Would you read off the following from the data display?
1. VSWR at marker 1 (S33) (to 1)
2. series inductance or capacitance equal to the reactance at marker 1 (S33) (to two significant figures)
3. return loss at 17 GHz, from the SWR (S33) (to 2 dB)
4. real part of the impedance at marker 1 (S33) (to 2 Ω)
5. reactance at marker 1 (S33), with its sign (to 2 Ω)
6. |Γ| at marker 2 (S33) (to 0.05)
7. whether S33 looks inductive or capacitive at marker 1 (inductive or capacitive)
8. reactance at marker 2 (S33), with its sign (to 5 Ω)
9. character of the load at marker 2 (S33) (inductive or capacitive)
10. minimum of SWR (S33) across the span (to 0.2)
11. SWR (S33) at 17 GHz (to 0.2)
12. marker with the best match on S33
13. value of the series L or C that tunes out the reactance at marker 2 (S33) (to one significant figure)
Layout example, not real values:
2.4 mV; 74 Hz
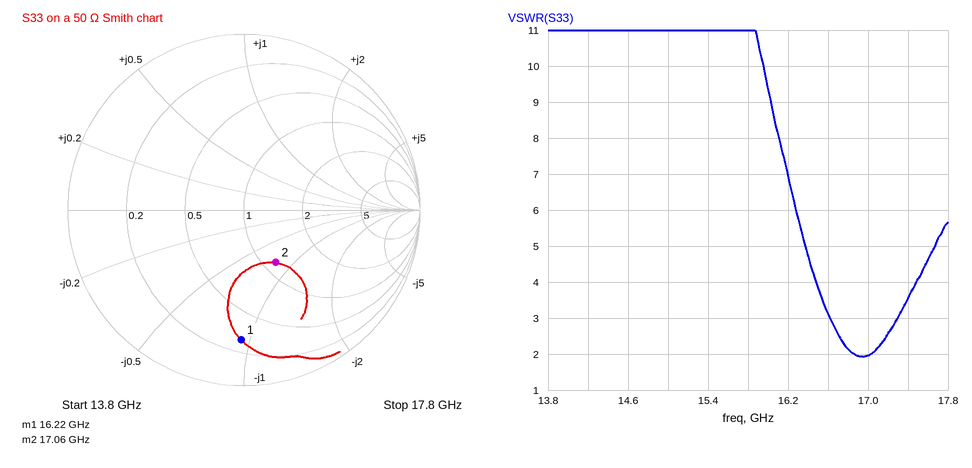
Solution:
7; 210 fF; 10 dB; 14 Ω; -46 Ω; 0.35; capacitive; -40 Ω; capacitive; 2.0; 2.0; marker 2; 400 pH
